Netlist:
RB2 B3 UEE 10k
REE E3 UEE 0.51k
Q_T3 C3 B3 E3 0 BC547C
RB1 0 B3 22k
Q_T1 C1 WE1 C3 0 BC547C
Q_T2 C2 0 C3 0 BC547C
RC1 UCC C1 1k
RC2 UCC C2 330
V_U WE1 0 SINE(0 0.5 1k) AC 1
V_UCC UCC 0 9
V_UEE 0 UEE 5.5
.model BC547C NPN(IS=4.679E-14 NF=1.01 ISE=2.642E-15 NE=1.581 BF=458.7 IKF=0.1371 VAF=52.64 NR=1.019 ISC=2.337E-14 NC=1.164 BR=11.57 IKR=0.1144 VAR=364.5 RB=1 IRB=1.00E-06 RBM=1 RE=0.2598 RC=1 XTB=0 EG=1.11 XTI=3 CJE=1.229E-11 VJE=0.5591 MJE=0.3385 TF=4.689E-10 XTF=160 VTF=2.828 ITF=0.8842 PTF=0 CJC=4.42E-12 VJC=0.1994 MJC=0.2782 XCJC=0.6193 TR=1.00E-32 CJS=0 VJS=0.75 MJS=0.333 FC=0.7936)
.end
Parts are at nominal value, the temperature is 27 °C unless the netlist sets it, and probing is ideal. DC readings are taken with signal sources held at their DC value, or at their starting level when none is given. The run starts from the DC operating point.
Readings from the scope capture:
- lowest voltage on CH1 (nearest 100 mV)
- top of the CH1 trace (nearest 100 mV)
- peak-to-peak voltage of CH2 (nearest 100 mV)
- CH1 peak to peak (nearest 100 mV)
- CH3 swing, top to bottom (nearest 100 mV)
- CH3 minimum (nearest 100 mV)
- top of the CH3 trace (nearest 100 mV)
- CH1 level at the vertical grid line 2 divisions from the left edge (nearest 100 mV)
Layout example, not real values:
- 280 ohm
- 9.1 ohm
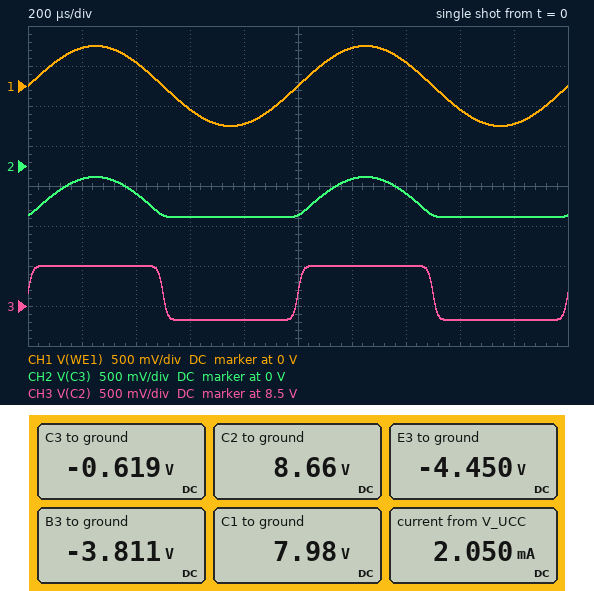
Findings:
- -500 mV
- 500 mV
- 500 mV
- 1.0 V
- 700 mV
- 8.3 V
- 9.0 V
- 300 mV
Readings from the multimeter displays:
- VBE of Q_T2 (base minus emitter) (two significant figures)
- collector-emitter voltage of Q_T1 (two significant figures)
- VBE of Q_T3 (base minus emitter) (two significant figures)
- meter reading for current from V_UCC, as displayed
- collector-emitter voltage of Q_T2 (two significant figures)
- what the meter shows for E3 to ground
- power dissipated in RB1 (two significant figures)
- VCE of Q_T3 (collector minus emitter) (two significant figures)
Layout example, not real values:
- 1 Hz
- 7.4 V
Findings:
- 620 mV
- 8.6 V
- 640 mV
- 2.050 mA
- 9.3 V
- -4.450 V
- 660 µW
- 3.8 V
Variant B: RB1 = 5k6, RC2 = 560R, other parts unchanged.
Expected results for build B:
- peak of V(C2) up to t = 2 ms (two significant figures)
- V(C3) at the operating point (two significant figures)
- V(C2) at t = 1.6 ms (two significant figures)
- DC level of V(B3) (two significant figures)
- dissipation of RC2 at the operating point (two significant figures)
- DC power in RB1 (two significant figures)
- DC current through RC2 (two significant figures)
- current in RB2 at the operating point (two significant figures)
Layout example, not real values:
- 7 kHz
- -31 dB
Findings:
- 9.0 V
- -650 mV
- 5.9 V
- -2.0 V
- 4.3 mW
- 730 µW
- 2.8 mA
- 350 µA
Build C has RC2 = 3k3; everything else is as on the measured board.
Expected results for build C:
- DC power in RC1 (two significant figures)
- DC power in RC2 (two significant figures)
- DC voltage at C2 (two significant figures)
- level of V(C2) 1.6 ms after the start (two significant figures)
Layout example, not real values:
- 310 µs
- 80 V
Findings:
- 1.1 mW
- 3.3 mW
- 5.7 V
- 2.2 V
